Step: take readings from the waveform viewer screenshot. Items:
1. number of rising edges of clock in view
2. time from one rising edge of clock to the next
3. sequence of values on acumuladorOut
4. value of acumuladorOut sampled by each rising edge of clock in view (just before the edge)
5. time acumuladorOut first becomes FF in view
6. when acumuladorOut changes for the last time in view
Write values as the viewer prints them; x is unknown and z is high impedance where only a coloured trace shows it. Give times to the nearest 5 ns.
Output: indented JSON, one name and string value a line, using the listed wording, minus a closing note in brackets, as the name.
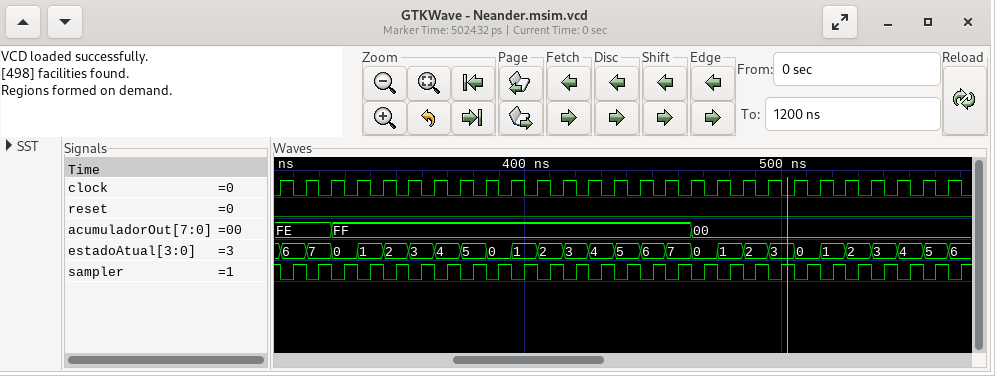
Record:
{
  "number of rising edges of clock in view": "27",
  "time from one rising edge of clock to the next": "10 ns",
  "sequence of values on acumuladorOut": "FE, FF, 00",
  "value of acumuladorOut sampled by each rising edge of clock in view": "FE, FE, FE, FF, FF, FF, FF, FF, FF, FF, FF, FF, FF, FF, FF, FF, FF, 00, 00, 00, 00, 00, 00, 00, 00, 00, 00",
  "time acumuladorOut first becomes FF in view": "325 ns",
  "when acumuladorOut changes for the last time in view": "465 ns"
}
